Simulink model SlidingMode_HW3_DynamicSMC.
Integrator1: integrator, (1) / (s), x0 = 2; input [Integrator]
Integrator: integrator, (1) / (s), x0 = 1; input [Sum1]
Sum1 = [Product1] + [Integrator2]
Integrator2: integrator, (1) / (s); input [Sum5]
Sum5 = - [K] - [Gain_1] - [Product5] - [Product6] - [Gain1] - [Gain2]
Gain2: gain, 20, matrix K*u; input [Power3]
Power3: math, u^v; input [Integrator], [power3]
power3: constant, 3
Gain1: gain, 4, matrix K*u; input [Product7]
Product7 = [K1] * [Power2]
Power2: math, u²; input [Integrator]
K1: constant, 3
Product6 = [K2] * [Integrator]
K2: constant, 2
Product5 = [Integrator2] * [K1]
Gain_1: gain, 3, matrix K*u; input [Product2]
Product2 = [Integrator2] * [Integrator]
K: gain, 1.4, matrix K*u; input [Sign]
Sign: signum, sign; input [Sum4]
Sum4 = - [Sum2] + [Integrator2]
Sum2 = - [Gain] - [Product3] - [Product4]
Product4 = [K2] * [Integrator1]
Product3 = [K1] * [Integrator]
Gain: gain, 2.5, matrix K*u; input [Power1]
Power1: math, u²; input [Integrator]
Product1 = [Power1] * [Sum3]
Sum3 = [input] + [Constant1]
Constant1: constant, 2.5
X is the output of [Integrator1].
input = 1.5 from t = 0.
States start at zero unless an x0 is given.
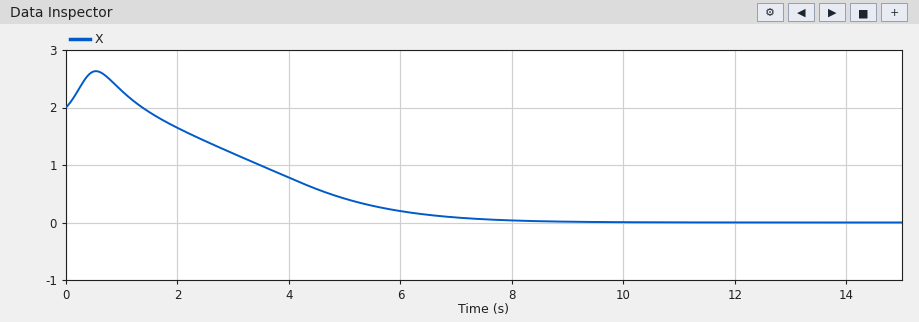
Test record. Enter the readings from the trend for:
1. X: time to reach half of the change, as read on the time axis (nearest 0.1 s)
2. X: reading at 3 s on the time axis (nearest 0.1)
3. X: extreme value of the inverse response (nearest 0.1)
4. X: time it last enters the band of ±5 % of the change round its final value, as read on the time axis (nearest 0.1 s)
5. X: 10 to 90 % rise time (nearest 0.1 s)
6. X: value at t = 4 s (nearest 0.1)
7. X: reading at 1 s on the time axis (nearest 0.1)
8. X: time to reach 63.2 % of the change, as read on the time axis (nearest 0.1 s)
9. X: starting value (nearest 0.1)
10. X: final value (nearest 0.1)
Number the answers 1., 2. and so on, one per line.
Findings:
1. 3.5 s
2. 1.2
3. 2.6
4. 6.8 s
5. 4.3 s
6. 0.8
7. 2.3
8. 4.1 s
9. 2.0
10. 0.0
